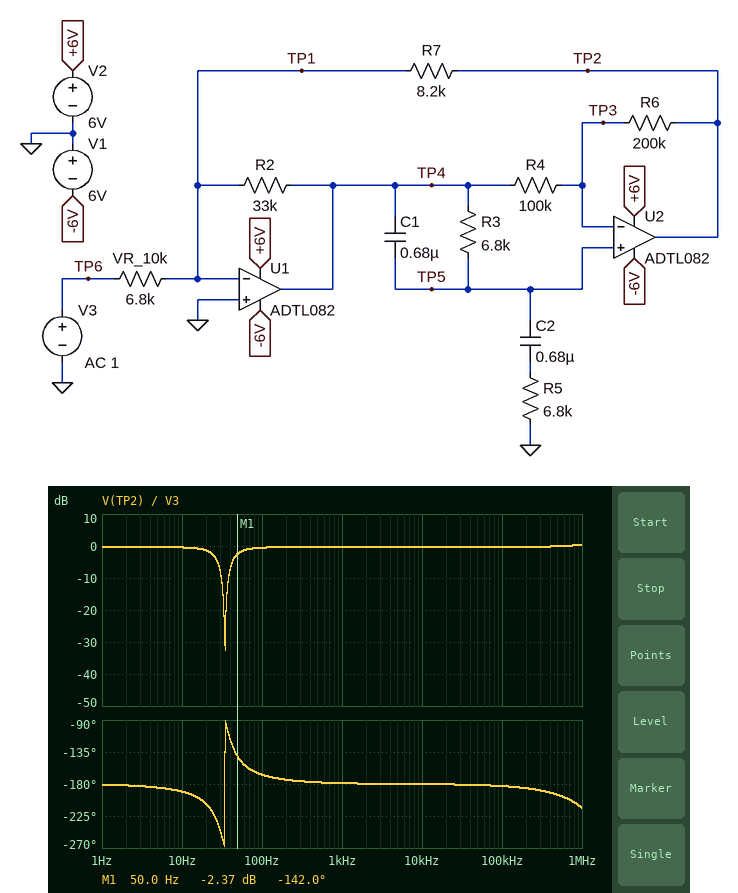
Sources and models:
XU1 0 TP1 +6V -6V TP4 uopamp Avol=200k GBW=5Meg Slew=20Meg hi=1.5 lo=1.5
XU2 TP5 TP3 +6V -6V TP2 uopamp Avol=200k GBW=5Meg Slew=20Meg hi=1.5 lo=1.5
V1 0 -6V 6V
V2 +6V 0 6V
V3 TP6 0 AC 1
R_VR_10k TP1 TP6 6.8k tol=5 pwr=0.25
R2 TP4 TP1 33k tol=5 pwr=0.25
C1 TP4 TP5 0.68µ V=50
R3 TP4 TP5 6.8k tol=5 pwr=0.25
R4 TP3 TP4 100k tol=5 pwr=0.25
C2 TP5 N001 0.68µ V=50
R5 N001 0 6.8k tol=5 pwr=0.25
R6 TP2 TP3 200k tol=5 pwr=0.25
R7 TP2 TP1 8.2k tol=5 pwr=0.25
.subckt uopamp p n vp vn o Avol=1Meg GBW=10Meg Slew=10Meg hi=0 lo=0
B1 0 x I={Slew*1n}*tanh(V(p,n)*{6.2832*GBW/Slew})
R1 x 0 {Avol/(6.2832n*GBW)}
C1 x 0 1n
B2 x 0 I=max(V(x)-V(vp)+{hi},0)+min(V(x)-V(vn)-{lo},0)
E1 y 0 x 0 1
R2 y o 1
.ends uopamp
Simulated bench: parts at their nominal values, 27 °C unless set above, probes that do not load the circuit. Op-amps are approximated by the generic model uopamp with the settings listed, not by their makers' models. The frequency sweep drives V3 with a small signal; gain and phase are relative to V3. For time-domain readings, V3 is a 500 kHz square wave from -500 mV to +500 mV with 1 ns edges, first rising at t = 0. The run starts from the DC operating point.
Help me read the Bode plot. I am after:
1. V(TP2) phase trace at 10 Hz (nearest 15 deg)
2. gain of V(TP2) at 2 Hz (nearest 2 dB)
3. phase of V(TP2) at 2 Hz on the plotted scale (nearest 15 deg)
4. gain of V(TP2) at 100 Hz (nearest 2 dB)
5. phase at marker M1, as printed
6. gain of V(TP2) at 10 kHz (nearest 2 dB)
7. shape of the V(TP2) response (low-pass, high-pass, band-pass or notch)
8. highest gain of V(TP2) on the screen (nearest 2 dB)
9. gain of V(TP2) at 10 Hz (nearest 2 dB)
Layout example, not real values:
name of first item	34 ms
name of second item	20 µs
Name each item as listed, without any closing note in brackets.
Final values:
V(TP2) phase trace at 10 Hz	-195 deg
gain of V(TP2) at 2 Hz	0 dB
phase of V(TP2) at 2 Hz on the plotted scale	-180 deg
gain of V(TP2) at 100 Hz	0 dB
phase at marker M1, as printed	-142.0 deg
gain of V(TP2) at 10 kHz	0 dB
shape of the V(TP2) response	notch
highest gain of V(TP2) on the screen	0 dB
gain of V(TP2) at 10 Hz	0 dB
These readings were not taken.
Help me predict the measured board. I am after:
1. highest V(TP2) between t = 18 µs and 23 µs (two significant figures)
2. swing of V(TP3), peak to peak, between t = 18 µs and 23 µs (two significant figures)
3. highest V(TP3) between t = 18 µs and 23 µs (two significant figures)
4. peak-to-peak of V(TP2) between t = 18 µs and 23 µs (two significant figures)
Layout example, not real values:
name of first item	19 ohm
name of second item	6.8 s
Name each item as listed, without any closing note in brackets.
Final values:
highest V(TP2) between t = 18 µs and 23 µs	620 mV
swing of V(TP3), peak to peak, between t = 18 µs and 23 µs	1.4 V
highest V(TP3) between t = 18 µs and 23 µs	690 mV
peak-to-peak of V(TP2) between t = 18 µs and 23 µs	1.2 V
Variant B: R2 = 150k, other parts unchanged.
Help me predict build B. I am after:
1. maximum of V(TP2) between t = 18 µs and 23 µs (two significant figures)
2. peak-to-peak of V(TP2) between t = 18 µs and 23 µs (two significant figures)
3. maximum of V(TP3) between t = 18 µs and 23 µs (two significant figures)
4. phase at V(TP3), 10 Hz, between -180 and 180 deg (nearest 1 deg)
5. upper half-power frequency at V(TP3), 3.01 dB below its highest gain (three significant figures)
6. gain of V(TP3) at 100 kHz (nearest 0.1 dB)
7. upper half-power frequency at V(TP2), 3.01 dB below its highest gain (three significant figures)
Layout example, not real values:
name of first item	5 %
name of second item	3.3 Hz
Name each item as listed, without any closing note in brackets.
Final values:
maximum of V(TP2) between t = 18 µs and 23 µs	790 mV
peak-to-peak of V(TP2) between t = 18 µs and 23 µs	1.6 V
maximum of V(TP3) between t = 18 µs and 23 µs	890 mV
phase at V(TP3), 10 Hz, between -180 and 180 deg	-150 deg
upper half-power frequency at V(TP3), 3.01 dB below its highest gain	37.2 Hz
gain of V(TP3) at 100 kHz	1.2 dB
upper half-power frequency at V(TP2), 3.01 dB below its highest gain	2.33 MHz
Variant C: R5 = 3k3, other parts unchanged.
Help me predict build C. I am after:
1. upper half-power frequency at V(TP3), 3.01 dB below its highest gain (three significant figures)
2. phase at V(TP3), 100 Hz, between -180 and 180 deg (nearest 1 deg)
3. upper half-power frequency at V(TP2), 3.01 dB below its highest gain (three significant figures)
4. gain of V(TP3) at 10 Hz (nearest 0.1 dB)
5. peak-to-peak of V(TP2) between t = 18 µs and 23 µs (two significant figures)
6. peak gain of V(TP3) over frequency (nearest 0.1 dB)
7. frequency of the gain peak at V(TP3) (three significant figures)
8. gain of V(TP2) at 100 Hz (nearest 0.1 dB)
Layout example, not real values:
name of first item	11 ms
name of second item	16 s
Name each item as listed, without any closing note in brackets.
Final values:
upper half-power frequency at V(TP3), 3.01 dB below its highest gain	52.4 Hz
phase at V(TP3), 100 Hz, between -180 and 180 deg	130 deg
upper half-power frequency at V(TP2), 3.01 dB below its highest gain	52.5 Hz
gain of V(TP3) at 10 Hz	0.5 dB
peak-to-peak of V(TP2) between t = 18 µs and 23 µs	1.2 V
peak gain of V(TP3) over frequency	24.8 dB
frequency of the gain peak at V(TP3)	49.4 Hz
gain of V(TP2) at 100 Hz	0.6 dB
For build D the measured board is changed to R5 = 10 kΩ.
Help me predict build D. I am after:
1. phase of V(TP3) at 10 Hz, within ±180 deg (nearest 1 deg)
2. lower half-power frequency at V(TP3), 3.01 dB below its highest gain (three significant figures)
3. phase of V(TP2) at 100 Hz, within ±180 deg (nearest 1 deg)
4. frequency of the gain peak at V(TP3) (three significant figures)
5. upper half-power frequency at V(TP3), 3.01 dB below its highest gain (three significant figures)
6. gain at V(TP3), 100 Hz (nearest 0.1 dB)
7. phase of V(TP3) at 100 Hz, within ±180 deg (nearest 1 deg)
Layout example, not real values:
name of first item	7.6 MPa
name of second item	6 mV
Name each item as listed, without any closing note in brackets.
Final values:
phase of V(TP3) at 10 Hz, within ±180 deg	-160 deg
lower half-power frequency at V(TP3), 3.01 dB below its highest gain	16.7 Hz
phase of V(TP2) at 100 Hz, within ±180 deg	-172 deg
frequency of the gain peak at V(TP3)	28.4 Hz
upper half-power frequency at V(TP3), 3.01 dB below its highest gain	48.3 Hz
gain at V(TP3), 100 Hz	0.8 dB
phase of V(TP3) at 100 Hz, within ±180 deg	163 deg
